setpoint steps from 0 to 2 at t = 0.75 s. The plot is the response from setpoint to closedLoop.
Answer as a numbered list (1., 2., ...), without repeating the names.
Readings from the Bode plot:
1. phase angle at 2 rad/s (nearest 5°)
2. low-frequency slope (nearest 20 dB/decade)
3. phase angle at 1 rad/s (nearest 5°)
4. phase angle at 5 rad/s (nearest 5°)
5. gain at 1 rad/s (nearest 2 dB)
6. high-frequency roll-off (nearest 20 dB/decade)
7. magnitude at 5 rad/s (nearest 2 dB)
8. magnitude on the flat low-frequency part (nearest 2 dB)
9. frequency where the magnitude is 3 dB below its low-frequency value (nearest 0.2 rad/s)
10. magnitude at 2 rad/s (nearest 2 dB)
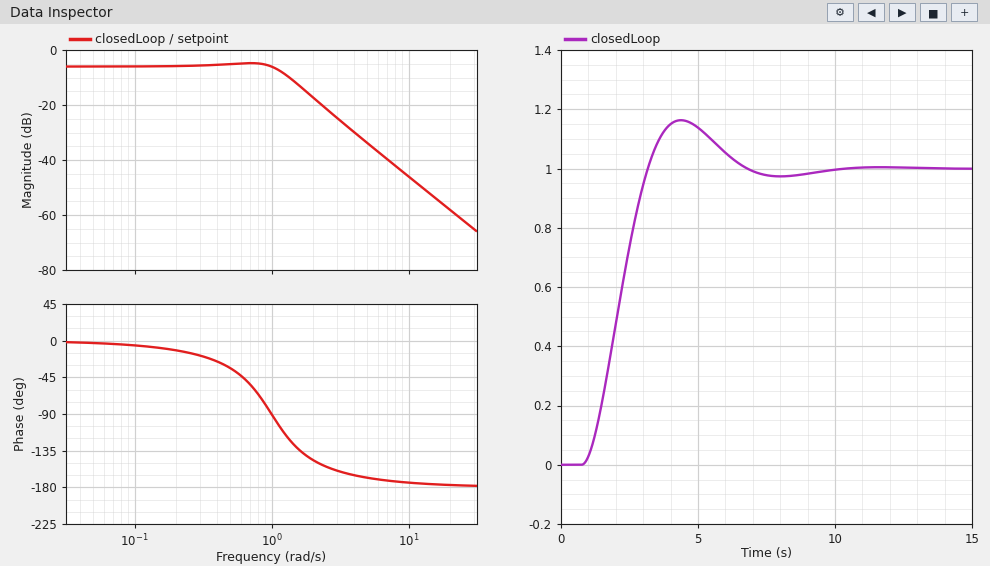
1. -145°
2. 0 dB/decade
3. -90°
4. -170°
5. -6 dB
6. -40 dB/decade
7. -34 dB
8. -6 dB
9. 1.2 rad/s
10. -18 dB
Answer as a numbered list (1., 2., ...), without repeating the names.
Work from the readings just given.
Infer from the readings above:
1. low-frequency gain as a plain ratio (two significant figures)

1. 0.50
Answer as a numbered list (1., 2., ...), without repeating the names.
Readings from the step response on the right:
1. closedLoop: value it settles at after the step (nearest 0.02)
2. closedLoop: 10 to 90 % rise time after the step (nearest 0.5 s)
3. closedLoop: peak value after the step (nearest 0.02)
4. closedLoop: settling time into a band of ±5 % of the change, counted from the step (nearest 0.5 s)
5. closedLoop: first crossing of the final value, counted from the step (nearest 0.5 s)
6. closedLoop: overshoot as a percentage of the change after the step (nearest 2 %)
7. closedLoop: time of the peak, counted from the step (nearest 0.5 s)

1. 1.00
2. 1.5 s
3. 1.16
4. 5.5 s
5. 2.5 s
6. 16 %
7. 3.5 s
